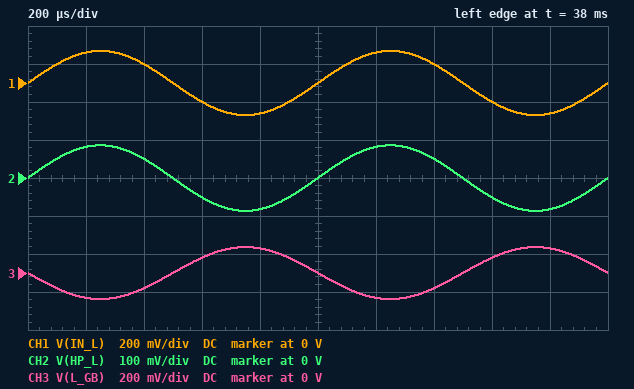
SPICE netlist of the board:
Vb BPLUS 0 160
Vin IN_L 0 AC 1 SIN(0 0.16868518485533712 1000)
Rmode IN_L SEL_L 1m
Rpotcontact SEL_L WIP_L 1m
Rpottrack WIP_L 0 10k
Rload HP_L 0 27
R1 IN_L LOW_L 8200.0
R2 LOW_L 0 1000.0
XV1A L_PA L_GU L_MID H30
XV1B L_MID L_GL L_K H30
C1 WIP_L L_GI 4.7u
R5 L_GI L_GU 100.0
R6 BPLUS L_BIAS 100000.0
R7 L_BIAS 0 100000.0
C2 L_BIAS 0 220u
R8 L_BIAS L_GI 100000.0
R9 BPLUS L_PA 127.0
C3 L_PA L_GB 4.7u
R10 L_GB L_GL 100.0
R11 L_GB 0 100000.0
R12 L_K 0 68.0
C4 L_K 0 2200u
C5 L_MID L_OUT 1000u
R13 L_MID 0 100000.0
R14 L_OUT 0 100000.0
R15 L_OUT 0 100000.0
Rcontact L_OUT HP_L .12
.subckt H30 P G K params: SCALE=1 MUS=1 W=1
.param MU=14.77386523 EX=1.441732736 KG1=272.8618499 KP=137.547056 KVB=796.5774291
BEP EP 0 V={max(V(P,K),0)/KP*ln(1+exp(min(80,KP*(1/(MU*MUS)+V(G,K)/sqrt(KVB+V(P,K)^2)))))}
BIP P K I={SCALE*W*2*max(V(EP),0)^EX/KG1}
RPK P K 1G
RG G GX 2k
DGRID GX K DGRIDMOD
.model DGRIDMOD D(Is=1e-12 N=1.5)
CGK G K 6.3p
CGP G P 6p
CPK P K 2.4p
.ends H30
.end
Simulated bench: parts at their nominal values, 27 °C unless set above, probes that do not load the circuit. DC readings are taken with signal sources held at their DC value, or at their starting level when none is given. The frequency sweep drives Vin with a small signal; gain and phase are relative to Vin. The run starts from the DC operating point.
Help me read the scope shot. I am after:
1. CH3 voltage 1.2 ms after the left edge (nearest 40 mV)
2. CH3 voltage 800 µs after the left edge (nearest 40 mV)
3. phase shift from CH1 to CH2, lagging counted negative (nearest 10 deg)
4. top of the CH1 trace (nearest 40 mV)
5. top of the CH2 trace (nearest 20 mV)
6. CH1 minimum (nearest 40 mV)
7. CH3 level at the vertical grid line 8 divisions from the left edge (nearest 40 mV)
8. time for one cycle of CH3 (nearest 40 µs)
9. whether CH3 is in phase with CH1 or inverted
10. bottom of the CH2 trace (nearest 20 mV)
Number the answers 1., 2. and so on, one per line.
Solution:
1. -120 mV
2. 120 mV
3. 0 deg
4. 160 mV
5. 80 mV
6. -160 mV
7. 80 mV
8. 1.00 ms
9. inverted
10. -80 mV
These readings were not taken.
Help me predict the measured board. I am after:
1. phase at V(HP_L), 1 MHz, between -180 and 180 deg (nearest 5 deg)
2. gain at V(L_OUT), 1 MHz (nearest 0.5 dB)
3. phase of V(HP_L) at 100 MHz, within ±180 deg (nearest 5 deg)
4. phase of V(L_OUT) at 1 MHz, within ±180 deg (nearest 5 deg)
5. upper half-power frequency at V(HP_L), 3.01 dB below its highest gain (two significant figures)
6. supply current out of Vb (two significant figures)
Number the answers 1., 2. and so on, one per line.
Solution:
1. 0 deg
2. -6.0 dB
3. -75 deg
4. 0 deg
5. 50 MHz
6. 38 mA
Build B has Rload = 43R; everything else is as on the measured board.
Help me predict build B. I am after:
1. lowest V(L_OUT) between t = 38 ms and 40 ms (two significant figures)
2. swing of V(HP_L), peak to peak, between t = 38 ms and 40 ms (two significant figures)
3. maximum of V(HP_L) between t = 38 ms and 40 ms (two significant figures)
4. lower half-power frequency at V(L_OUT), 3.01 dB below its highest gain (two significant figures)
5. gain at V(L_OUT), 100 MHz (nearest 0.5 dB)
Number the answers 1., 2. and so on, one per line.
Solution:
1. -100 mV
2. 210 mV
3. 100 mV
4. 2.9 Hz
5. -13.0 dB
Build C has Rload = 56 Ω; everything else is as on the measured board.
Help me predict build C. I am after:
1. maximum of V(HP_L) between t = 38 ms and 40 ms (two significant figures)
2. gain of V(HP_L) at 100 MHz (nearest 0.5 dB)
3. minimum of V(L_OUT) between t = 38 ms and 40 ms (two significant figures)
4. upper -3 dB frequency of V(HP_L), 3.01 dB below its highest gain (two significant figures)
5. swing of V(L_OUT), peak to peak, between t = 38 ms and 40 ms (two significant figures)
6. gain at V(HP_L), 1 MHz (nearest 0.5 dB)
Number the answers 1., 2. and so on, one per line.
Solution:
1. 110 mV
2. -11.5 dB
3. -110 mV
4. 60 MHz
5. 220 mV
6. -3.5 dB
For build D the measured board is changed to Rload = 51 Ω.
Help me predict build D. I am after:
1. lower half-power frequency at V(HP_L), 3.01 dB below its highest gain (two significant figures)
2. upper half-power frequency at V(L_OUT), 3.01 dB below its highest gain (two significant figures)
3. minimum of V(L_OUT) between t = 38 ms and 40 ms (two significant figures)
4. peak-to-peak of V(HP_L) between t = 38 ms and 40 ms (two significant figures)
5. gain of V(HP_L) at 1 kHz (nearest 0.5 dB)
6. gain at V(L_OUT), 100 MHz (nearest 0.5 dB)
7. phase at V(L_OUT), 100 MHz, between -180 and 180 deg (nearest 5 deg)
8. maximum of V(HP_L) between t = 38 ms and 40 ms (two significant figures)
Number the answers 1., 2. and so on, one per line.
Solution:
1. 2.6 Hz
2. 59 MHz
3. -110 mV
4. 220 mV
5. -4.0 dB
6. -12.0 dB
7. -75 deg
8. 110 mV
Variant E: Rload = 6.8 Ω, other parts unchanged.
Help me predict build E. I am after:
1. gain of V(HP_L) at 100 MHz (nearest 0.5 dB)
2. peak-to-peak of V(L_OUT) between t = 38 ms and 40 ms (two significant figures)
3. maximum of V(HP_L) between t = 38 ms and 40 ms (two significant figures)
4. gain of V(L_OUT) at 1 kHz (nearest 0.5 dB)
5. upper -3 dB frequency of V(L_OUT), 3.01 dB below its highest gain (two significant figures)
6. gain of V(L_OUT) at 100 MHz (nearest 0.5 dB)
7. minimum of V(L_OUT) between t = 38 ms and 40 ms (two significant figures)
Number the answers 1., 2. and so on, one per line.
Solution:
1. -25.5 dB
2. 76 mV
3. 37 mV
4. -13.0 dB
5. 38 MHz
6. -25.0 dB
7. -38 mV
